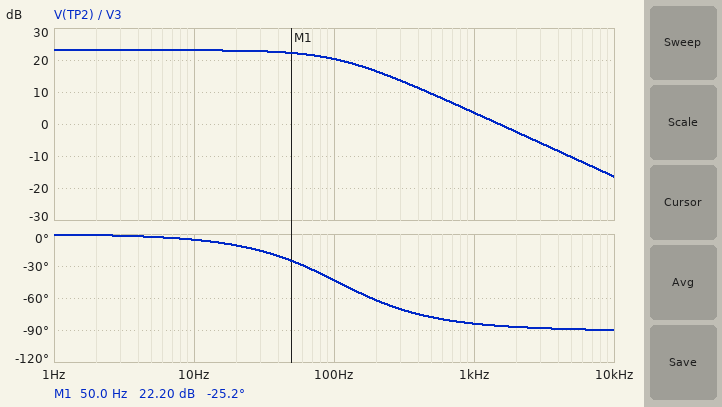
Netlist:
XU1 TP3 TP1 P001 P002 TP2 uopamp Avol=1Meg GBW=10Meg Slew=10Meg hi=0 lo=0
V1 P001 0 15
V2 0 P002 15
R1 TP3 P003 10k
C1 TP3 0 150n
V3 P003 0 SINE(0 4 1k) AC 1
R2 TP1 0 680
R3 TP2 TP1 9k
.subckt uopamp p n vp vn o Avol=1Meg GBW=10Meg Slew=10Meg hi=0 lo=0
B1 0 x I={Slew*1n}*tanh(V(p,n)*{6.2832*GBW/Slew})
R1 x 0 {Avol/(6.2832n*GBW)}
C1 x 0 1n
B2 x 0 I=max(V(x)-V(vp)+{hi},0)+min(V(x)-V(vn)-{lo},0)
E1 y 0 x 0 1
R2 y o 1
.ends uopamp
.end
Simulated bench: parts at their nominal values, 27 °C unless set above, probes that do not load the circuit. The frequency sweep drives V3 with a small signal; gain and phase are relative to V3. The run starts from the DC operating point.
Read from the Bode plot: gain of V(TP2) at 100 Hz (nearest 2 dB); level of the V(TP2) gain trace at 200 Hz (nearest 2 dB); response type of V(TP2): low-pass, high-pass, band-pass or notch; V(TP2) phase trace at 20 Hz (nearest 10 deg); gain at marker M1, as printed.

20 dB
16 dB
low-pass
-10 deg
22.20 dB
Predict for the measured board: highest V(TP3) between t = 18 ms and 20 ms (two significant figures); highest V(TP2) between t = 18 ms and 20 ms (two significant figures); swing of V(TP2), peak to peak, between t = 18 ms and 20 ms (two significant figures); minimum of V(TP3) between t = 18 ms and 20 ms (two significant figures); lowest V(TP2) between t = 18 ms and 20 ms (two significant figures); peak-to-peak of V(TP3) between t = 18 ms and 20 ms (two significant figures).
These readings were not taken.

420 mV
6.0 V
12 V
-420 mV
-6.0 V
840 mV
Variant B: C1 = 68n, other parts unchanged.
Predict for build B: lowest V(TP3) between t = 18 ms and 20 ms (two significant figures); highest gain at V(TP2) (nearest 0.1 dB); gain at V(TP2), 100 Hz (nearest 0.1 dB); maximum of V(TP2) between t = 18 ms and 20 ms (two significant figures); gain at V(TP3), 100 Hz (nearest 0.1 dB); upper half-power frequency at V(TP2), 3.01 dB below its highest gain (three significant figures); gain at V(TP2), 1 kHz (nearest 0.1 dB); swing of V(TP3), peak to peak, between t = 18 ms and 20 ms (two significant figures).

-910 mV
23.1 dB
22.3 dB
13 V
-0.7 dB
234 Hz
10.2 dB
1.8 V
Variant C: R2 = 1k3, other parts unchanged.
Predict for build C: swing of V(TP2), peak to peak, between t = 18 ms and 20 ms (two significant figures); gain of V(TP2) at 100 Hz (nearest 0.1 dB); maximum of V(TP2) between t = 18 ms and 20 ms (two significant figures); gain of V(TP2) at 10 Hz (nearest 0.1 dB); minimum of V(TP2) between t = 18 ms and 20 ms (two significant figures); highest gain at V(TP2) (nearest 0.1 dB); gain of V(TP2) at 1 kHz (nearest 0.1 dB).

6.7 V
15.2 dB
3.3 V
17.9 dB
-3.3 V
18.0 dB
-1.6 dB
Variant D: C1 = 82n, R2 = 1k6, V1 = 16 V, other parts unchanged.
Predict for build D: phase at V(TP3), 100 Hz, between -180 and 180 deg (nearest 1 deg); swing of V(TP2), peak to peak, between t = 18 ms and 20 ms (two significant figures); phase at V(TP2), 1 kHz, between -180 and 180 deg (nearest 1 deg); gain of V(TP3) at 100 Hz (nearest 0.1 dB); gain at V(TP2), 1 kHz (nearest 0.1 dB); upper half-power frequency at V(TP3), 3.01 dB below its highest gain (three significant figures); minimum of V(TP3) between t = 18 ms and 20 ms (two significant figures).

-27 deg
10 V
-79 deg
-1.0 dB
2.0 dB
194 Hz
-760 mV
